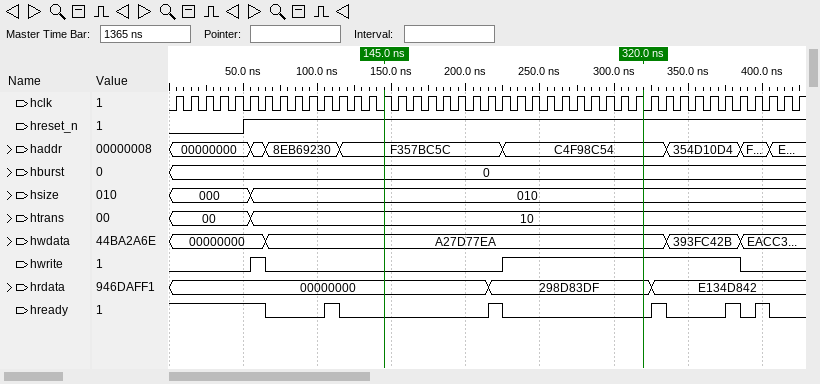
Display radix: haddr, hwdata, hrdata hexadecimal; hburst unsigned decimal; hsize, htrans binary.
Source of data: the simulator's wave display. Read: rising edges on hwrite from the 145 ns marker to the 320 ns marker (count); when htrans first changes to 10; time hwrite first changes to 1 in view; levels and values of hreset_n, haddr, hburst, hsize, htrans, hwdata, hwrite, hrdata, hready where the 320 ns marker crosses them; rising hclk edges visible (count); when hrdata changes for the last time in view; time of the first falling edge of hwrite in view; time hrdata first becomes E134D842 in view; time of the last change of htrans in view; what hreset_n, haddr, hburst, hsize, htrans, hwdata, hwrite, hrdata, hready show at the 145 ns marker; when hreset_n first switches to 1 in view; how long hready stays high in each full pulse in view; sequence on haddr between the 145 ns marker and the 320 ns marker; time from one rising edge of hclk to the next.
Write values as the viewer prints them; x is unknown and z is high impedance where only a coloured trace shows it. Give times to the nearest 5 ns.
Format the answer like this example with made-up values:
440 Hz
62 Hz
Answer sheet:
1
55 ns
55 ns
hreset_n=1, haddr=C4F98C54, hburst=0, hsize=010, htrans=10, hwdata=A27D77EA, hwrite=1, hrdata=298D83DF, hready=0
43
325 ns
65 ns
325 ns
55 ns
hreset_n=1, haddr=F357BC5C, hburst=0, hsize=010, htrans=10, hwdata=A27D77EA, hwrite=0, hrdata=00000000, hready=0
50 ns
10 ns, 10 ns, 10 ns, 10 ns, 10 ns
F357BC5C, C4F98C54
10 ns
